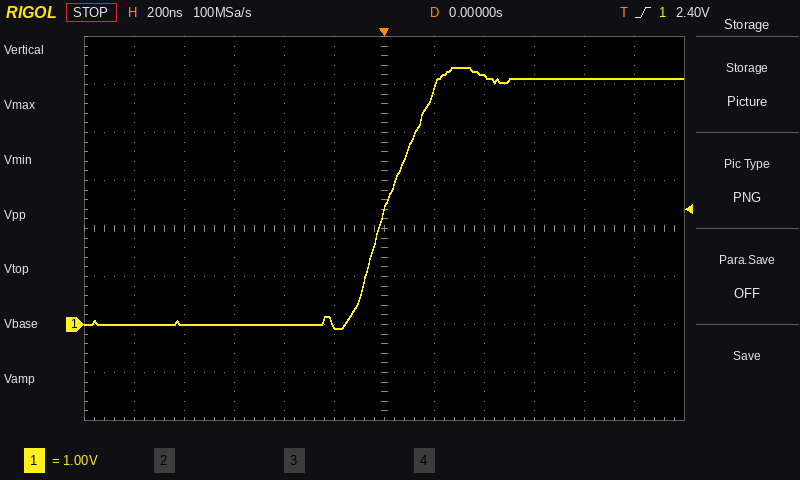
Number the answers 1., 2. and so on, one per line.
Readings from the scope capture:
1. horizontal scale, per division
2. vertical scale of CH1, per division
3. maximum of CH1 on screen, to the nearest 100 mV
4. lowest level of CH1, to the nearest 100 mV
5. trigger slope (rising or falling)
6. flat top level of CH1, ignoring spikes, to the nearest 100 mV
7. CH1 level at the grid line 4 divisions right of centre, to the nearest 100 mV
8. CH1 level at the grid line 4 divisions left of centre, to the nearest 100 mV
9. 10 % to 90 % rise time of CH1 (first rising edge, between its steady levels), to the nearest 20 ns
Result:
1. 200 ns
2. 1 V
3. 5.4 V
4. -100 mV
5. rising
6. 5.1 V
7. 5.1 V
8. 0.0 V
9. 280 ns
